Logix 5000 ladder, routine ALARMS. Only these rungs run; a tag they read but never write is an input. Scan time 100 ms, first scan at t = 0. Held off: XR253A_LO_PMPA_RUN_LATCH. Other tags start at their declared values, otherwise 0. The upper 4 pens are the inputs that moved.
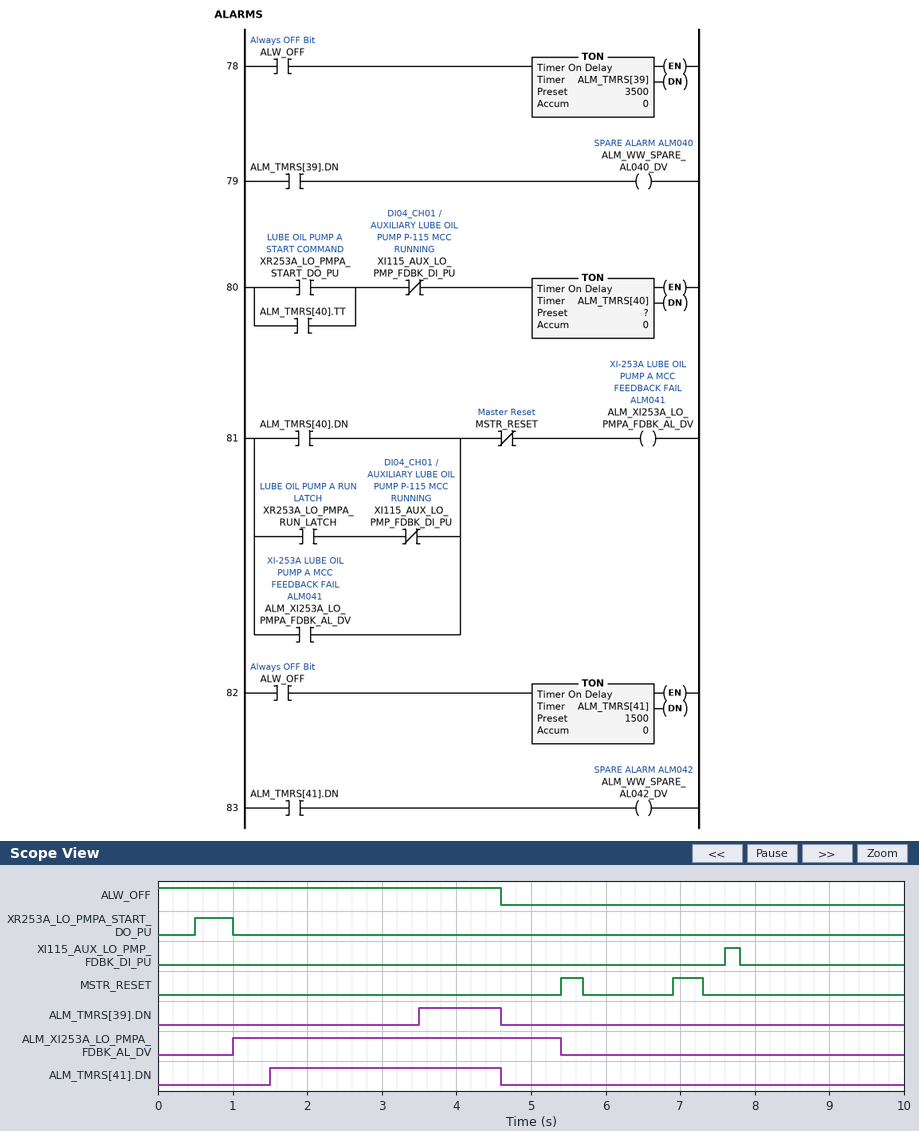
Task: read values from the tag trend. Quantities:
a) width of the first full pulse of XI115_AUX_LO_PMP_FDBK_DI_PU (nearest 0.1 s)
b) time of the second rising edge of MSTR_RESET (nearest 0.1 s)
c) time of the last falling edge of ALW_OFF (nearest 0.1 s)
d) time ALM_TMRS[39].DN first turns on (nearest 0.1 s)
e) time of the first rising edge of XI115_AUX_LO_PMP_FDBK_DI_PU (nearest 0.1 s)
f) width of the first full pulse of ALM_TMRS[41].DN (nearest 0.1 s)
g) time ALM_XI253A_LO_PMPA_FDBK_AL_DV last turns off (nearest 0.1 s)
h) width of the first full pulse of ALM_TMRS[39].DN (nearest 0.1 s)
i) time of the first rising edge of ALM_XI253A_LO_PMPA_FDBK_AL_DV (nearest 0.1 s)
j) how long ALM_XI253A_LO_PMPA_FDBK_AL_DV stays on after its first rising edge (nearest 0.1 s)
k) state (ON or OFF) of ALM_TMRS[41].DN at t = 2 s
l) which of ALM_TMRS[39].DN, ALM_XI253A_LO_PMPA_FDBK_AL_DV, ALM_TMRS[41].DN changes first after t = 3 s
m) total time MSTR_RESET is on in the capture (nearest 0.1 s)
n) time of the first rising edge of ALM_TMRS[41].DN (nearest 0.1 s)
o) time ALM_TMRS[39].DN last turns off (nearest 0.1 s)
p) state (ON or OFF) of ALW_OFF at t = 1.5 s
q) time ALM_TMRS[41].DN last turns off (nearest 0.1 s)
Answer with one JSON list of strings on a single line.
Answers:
["0.2 s", "6.9 s", "4.6 s", "3.5 s", "7.6 s", "3.1 s", "5.4 s", "1.1 s", "1.0 s", "4.4 s", "ON", "ALM_TMRS[39].DN", "0.7 s", "1.5 s", "4.6 s", "ON", "4.6 s"]
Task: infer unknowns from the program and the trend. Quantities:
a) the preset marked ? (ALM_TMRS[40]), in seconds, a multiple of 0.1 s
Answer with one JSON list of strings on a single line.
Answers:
["0.5 s"]
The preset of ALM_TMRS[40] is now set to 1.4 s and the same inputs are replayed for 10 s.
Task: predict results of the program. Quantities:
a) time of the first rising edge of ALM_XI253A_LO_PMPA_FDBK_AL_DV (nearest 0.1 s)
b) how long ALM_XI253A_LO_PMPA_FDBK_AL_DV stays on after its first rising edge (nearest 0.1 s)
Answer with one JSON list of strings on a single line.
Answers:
["1.9 s", "3.5 s"]
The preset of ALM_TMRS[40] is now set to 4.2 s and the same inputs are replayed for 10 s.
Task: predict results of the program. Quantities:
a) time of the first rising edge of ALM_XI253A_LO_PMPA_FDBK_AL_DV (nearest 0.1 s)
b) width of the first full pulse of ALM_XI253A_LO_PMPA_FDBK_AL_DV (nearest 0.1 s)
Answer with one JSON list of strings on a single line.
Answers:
["4.7 s", "0.7 s"]
